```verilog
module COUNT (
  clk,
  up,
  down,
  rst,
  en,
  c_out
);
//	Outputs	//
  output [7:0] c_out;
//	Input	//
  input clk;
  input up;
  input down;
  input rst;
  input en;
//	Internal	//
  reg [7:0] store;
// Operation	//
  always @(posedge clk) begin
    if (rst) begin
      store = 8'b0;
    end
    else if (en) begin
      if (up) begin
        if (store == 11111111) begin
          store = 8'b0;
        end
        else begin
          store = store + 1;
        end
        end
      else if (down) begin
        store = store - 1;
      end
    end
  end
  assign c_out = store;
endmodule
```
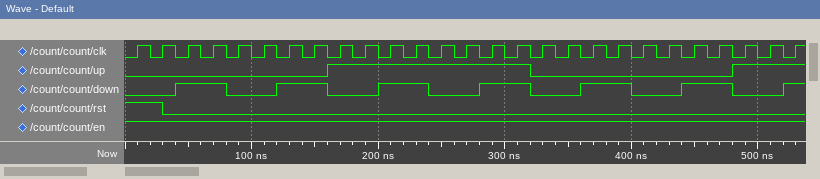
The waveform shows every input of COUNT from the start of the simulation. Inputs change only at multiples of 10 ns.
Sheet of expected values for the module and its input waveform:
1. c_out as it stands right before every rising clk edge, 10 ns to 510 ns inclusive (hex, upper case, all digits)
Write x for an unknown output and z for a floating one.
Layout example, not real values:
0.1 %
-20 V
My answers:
x, 00, 00, FF, FE, FE, FE, FD, FC, FD, FE, FF, 00, 01, 02, 03, 04, 04, 04, 03, 02, 02, 02, 01, 00, 01
